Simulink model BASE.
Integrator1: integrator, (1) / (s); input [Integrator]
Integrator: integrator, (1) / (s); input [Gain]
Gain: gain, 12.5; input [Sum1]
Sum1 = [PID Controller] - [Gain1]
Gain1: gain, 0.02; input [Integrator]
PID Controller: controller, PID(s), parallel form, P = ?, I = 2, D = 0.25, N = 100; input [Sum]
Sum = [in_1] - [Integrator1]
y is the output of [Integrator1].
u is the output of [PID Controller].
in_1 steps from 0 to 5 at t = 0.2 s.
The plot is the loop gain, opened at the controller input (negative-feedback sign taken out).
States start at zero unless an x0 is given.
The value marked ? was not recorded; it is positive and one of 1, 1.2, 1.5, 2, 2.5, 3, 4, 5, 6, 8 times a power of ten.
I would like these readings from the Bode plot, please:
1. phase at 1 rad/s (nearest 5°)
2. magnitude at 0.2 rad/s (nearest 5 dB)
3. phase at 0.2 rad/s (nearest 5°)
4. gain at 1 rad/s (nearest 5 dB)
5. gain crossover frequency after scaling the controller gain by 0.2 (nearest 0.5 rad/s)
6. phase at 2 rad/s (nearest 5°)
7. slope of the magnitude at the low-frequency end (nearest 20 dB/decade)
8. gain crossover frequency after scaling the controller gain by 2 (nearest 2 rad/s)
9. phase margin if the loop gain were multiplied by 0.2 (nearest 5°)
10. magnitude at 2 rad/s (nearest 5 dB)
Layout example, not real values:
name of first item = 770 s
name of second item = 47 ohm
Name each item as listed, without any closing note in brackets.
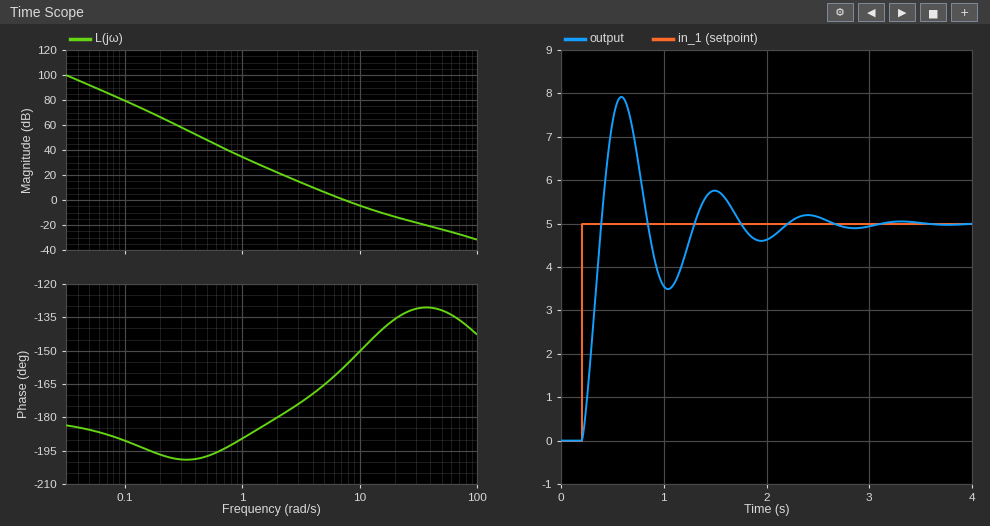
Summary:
phase at 1 rad/s = -190°
magnitude at 0.2 rad/s = 65 dB
phase at 0.2 rad/s = -195°
gain at 1 rad/s = 35 dB
gain crossover frequency after scaling the controller gain by 0.2 = 3.0 rad/s
phase at 2 rad/s = -180°
slope of the magnitude at the low-frequency end = -40 dB/decade
gain crossover frequency after scaling the controller gain by 2 = 12 rad/s
phase margin if the loop gain were multiplied by 0.2 = 5°
magnitude at 2 rad/s = 20 dB
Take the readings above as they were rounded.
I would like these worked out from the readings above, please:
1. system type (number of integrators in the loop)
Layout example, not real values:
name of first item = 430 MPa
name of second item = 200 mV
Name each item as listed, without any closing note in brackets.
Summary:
system type = 2
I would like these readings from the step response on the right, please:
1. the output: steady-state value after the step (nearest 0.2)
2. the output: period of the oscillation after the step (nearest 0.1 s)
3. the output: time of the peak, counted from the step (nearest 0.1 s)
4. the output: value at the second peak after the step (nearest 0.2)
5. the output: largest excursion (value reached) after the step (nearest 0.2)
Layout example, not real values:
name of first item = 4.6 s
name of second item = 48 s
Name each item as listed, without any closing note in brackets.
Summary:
the output: steady-state value after the step = 5.0
the output: period of the oscillation after the step = 0.9 s
the output: time of the peak, counted from the step = 0.4 s
the output: value at the second peak after the step = 5.8
the output: largest excursion (value reached) after the step = 8.0
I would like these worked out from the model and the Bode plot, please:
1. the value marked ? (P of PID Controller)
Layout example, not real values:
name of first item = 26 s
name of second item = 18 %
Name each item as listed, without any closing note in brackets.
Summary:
the value marked ? = 4
